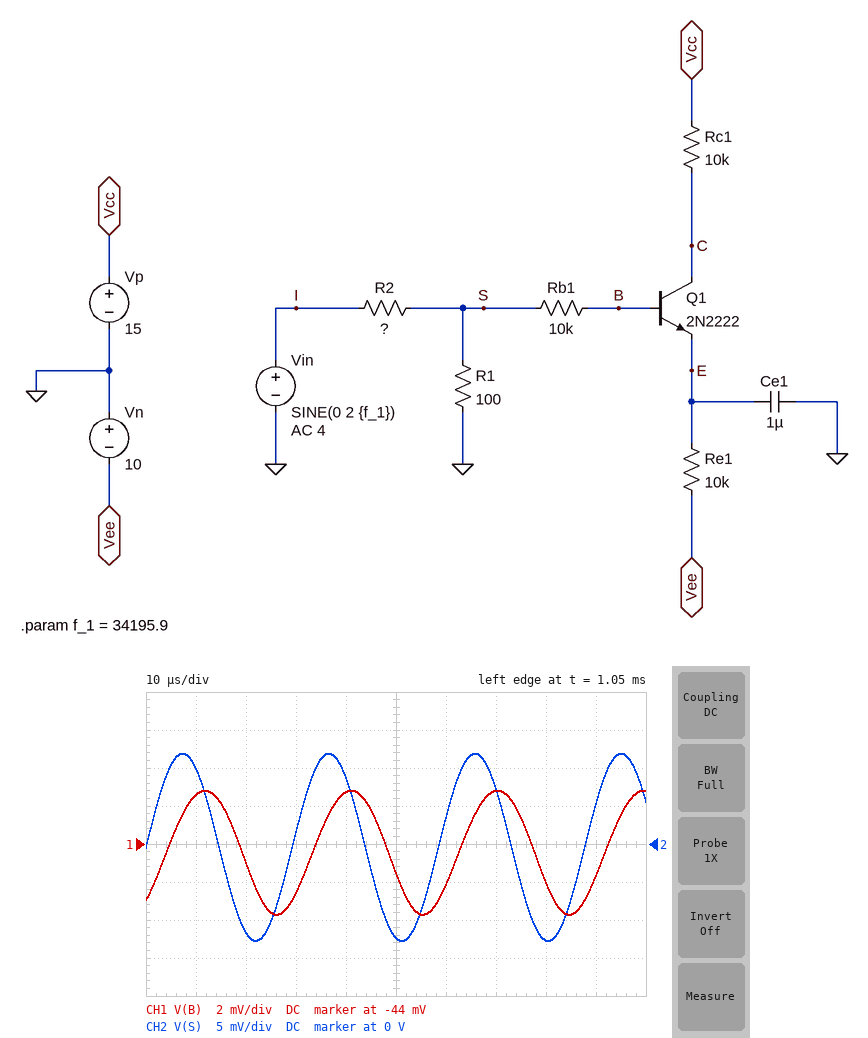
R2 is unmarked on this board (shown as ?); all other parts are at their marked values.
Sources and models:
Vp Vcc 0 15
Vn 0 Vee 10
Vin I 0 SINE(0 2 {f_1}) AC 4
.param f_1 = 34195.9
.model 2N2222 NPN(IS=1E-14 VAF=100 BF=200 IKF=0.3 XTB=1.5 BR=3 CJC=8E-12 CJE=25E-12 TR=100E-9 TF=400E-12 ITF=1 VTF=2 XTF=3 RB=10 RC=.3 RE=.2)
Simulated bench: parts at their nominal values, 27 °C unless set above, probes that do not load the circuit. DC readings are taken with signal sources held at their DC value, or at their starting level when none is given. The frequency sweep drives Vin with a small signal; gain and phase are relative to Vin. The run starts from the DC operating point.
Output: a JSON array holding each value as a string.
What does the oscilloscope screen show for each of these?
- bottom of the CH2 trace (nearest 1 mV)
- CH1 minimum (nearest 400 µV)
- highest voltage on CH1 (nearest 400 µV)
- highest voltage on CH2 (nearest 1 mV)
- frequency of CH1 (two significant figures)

["-13 mV", "-47.6 mV", "-41.2 mV", "12 mV", "34 kHz"]
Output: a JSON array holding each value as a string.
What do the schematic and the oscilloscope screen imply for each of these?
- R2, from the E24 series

["16 kΩ"]
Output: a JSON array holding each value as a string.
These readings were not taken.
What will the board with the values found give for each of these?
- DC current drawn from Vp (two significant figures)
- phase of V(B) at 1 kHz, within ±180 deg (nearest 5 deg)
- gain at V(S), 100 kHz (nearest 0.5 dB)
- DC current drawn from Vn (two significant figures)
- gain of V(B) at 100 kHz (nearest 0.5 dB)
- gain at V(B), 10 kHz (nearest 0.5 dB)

["930 µA", "-15 deg", "-44.0 dB", "930 µA", "-63.0 dB", "-52.0 dB"]
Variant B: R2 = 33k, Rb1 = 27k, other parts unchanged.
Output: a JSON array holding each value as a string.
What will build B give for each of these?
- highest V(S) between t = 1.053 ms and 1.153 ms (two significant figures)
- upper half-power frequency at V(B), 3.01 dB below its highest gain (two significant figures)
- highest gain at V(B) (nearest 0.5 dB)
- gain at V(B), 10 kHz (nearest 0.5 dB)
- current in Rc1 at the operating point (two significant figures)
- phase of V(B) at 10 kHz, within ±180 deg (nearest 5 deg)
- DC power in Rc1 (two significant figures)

["5.6 mV", "1.0 kHz", "-50.5 dB", "-64.5 dB", "920 µA", "-45 deg", "8.4 mW"]
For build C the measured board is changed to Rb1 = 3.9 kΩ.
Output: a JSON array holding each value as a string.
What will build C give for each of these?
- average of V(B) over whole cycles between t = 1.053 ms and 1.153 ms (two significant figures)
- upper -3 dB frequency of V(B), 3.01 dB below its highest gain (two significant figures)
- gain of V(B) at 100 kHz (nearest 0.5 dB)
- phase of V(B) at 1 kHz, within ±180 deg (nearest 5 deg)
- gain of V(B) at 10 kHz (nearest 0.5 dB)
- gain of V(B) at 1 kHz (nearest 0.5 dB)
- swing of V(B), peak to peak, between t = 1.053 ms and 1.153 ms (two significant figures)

["-18 mV", "7.3 kHz", "-55.5 dB", "-5 deg", "-47.5 dB", "-44.5 dB", "13 mV"]
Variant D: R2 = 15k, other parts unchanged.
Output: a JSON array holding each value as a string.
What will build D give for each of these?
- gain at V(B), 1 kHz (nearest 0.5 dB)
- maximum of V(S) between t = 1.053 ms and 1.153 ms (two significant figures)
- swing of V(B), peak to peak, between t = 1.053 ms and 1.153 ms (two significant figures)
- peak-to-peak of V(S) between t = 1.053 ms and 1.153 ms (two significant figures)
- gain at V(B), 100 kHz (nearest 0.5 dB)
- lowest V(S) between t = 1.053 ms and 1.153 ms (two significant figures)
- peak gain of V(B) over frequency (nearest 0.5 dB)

["-44.5 dB", "13 mV", "7.0 mV", "26 mV", "-62.5 dB", "-14 mV", "-43.5 dB"]
